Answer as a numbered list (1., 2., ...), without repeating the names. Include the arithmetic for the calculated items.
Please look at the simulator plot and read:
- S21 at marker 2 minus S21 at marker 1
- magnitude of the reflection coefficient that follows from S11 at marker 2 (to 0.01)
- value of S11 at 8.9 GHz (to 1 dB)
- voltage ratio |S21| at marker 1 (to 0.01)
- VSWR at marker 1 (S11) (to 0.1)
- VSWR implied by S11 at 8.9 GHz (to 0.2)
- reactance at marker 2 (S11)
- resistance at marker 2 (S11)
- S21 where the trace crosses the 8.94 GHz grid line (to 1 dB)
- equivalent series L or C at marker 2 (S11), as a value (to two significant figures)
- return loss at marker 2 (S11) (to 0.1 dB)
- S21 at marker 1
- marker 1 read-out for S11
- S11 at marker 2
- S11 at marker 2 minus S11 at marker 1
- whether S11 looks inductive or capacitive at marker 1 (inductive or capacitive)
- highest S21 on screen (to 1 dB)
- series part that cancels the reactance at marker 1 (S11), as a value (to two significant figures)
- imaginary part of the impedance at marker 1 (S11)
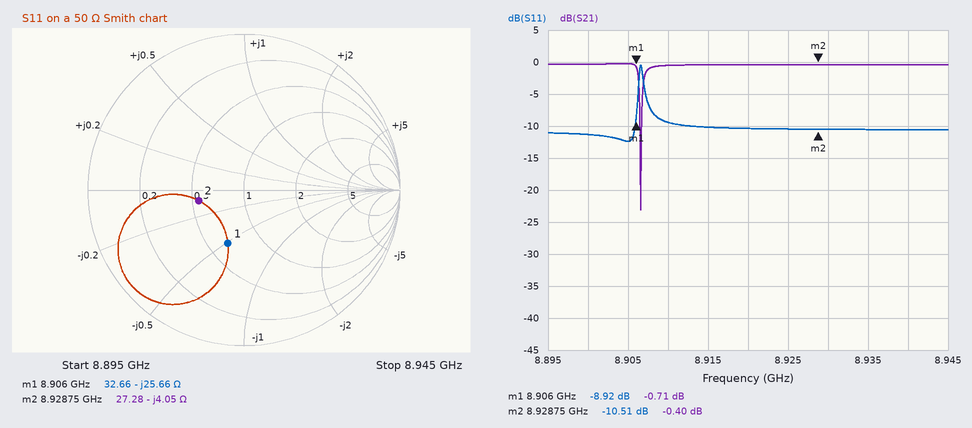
1. -0.4 − (-0.71) = 0.31 dB
2. 10^(-10.51/20) ≈ 0.30
3. -11 dB
4. 10^(-0.71/20) ≈ 0.92
5. 2.1
6. |Γ| = 10^(-11/20) = 0.2818; VSWR = (1 + 0.2818)/(1 − 0.2818) ≈ 1.8
7. -4.05 Ω
8. 27.28 Ω
9. 0 dB
10. C = 1/(2π × 8.92875 GHz × 4.05 Ω) ≈ 4.4 pF
11. 10.5 dB
12. -0.71 dB
13. -8.92 dB
14. -10.51 dB
15. -10.51 − (-8.92) = -1.59 dB
16. capacitive
17. 0 dB
18. L = 25.66 Ω/(2π × 8.906 GHz) ≈ 459 pH, so 460 pH to two significant figures
19. -25.66 Ω
